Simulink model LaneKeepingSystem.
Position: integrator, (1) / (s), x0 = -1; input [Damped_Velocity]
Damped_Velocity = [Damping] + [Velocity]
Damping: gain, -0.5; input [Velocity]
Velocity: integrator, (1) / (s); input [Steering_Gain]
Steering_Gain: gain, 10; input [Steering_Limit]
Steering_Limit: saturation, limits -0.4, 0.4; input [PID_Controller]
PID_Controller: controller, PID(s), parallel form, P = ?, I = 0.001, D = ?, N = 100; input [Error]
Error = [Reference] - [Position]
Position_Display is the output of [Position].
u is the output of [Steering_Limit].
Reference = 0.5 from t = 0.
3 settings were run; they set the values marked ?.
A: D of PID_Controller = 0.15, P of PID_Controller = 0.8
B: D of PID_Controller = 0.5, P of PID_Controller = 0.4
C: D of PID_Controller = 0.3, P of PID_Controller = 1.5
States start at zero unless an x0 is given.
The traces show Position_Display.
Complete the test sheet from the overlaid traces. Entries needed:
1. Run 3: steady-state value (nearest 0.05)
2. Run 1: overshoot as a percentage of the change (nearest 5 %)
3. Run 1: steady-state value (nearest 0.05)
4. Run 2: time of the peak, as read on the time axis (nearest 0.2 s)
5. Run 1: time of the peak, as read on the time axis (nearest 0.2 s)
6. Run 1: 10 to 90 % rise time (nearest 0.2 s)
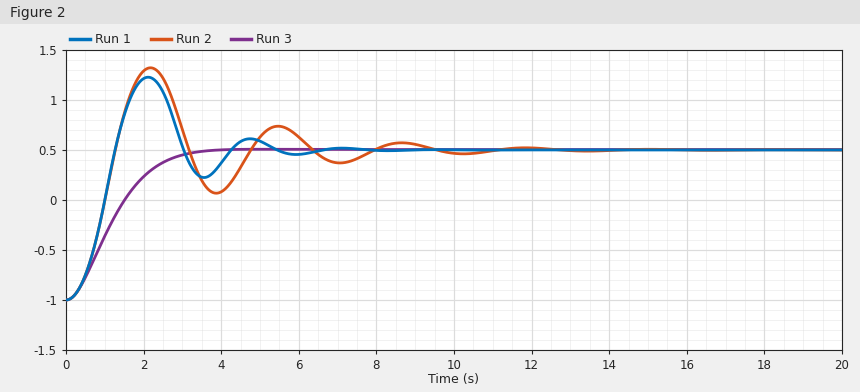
0.50
50 %
0.50
2.2 s
2.2 s
0.8 s
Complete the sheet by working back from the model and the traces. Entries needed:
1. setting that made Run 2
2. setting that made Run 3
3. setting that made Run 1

A
B
C
